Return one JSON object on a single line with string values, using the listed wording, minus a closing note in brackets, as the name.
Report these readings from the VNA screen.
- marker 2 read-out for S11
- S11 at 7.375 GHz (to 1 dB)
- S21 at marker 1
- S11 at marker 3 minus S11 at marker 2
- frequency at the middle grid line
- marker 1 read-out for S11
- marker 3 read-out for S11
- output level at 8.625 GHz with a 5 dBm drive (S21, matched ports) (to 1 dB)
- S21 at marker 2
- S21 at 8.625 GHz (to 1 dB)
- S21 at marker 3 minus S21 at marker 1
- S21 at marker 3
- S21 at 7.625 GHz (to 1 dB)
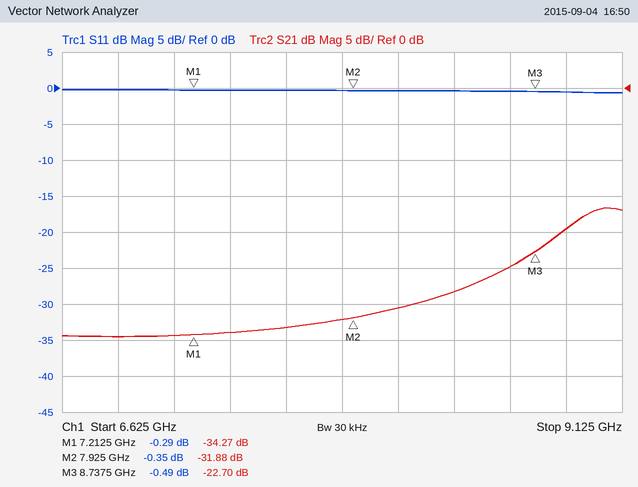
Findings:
{"marker 2 read-out for S11": "-0.35 dB", "S11 at 7.375 GHz": "0 dB", "S21 at marker 1": "-34.27 dB", "S11 at marker 3 minus S11 at marker 2": "-0.14 dB", "frequency at the middle grid line": "7.875 GHz", "marker 1 read-out for S11": "-0.29 dB", "marker 3 read-out for S11": "-0.49 dB", "output level at 8.625 GHz with a 5 dBm drive (S21, matched ports)": "-20 dBm", "S21 at marker 2": "-31.88 dB", "S21 at 8.625 GHz": "-25 dB", "S21 at marker 3 minus S21 at marker 1": "11.57 dB", "S21 at marker 3": "-22.70 dB", "S21 at 7.625 GHz": "-33 dB"}
